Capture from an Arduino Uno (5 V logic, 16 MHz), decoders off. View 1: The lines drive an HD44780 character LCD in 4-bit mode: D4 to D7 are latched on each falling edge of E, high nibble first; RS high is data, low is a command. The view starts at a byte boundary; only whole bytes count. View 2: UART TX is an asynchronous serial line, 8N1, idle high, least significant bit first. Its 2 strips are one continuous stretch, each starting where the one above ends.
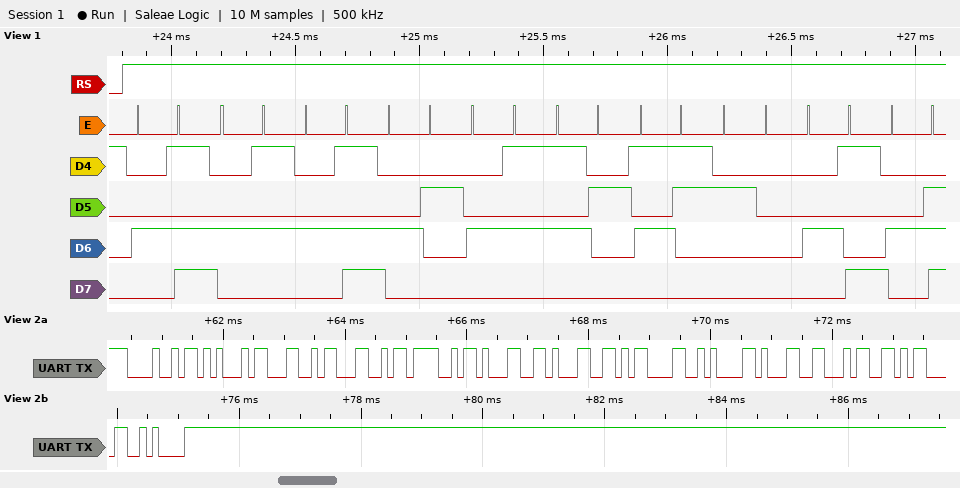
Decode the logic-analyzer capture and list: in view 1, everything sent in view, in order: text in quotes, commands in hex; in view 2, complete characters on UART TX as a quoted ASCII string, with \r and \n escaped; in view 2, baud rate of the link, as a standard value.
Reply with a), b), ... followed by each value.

a) "MEMBERS IN"
b) "HELLO11\r\n14\r\n"
c) 9600 baud
